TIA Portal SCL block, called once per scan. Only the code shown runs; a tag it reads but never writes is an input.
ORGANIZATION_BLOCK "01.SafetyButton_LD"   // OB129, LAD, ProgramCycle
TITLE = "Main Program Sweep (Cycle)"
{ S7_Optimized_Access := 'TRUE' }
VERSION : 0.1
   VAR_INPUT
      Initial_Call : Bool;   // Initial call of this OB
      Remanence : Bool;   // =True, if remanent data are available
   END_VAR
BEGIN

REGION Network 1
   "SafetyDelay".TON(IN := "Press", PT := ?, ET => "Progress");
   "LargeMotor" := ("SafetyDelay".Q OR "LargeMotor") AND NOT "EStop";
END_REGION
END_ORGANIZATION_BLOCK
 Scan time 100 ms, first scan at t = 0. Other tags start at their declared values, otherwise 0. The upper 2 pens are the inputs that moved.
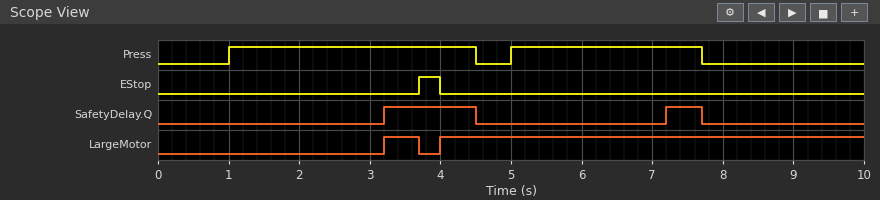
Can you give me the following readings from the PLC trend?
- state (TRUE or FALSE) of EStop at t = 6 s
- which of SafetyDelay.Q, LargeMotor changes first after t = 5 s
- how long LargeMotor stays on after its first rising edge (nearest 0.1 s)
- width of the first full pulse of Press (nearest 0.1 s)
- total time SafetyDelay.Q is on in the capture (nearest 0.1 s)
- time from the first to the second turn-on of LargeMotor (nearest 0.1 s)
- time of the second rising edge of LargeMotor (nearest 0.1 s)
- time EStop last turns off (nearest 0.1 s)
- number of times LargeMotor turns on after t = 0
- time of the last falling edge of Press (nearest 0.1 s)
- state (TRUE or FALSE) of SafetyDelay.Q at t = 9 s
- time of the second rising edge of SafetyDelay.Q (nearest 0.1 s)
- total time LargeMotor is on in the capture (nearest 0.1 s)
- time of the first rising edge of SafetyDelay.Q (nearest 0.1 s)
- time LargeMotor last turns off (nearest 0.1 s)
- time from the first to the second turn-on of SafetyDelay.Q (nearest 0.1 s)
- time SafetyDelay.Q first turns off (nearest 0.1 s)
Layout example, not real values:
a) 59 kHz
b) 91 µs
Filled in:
a) FALSE
b) SafetyDelay.Q
c) 0.5 s
d) 3.5 s
e) 1.8 s
f) 0.8 s
g) 4.0 s
h) 4.0 s
i) 2
j) 7.7 s
k) FALSE
l) 7.2 s
m) 6.5 s
n) 3.2 s
o) 3.7 s
p) 4.0 s
q) 4.5 s
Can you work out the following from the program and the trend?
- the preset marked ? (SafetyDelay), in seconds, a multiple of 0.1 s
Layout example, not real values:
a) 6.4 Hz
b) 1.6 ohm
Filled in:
a) 2.2 s
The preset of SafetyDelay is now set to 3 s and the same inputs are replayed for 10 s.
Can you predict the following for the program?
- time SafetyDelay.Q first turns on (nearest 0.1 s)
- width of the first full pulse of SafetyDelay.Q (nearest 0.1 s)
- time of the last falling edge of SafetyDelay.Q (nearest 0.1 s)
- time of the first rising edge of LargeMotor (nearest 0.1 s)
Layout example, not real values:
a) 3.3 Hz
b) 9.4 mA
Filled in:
a) 4.0 s
b) 0.5 s
c) 4.5 s
d) 4.0 s
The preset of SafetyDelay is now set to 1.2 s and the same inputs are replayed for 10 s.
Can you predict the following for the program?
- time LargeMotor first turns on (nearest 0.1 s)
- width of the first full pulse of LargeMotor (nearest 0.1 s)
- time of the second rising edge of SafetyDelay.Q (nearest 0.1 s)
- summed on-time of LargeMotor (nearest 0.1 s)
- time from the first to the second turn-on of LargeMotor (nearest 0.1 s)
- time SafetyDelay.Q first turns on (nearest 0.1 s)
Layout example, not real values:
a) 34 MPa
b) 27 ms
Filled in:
a) 2.2 s
b) 1.5 s
c) 6.2 s
d) 7.5 s
e) 1.8 s
f) 2.2 s
